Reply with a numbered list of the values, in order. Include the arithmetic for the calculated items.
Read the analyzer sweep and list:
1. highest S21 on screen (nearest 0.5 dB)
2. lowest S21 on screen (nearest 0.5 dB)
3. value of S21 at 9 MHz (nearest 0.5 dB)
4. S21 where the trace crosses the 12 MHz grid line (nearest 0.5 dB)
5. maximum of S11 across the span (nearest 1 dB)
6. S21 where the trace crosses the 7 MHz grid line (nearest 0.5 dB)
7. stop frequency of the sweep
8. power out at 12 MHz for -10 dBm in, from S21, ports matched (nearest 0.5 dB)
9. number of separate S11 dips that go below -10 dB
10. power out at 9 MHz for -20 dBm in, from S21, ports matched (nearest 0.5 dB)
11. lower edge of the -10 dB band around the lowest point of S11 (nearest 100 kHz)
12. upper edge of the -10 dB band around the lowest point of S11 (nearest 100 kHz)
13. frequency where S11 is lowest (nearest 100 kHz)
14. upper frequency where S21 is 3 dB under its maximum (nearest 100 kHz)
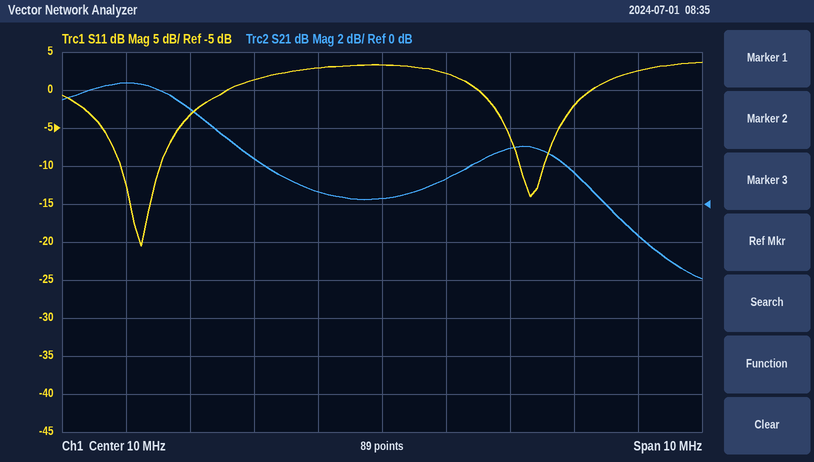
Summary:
1. 6.5 dB
2. -4.0 dB
3. 0.5 dB
4. 3.0 dB
5. 4 dB
6. 5.0 dB
7. 15 MHz
8. -10 dBm + (3.0 dB) = -7.0 dBm
9. 2
10. -20 dBm + (0.5 dB) = -19.5 dBm
11. 5.9 MHz
12. 6.5 MHz
13. 6.2 MHz
14. 7.6 MHz
